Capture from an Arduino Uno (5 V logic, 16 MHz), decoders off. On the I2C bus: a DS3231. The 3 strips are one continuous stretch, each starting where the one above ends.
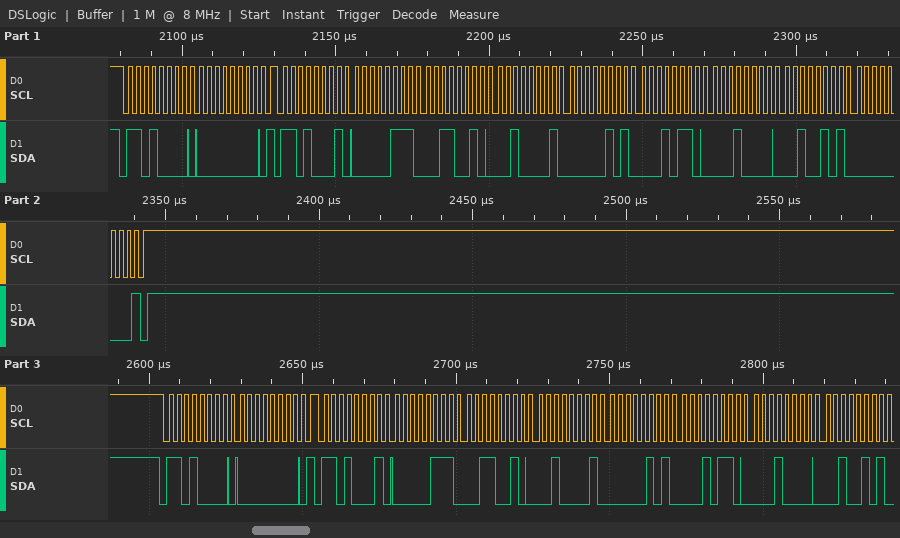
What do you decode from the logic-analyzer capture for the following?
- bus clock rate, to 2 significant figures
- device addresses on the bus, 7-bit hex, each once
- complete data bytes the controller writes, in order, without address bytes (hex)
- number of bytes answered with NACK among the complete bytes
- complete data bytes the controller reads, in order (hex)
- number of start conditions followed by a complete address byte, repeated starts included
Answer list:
400 kHz
0x68
00 00
1
07 32 21 05 16 10 25 00 07 32 21 05 16 10 25
4
